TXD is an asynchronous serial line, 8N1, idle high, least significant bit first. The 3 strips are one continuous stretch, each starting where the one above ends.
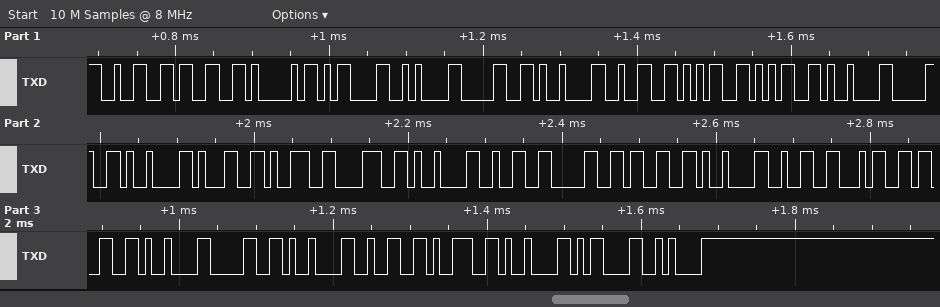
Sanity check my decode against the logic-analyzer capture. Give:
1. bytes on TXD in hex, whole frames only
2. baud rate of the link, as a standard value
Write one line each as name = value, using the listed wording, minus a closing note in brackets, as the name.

bytes on TXD in hex, whole frames only = 32 33 41 0D 0A 30 09 32 35 35 09 30 09 31 39 38 09 32 30 33 09 32 34 33 09 30 09 32 39 09 0D 0A
baud rate of the link, as a standard value = 115200 baud
